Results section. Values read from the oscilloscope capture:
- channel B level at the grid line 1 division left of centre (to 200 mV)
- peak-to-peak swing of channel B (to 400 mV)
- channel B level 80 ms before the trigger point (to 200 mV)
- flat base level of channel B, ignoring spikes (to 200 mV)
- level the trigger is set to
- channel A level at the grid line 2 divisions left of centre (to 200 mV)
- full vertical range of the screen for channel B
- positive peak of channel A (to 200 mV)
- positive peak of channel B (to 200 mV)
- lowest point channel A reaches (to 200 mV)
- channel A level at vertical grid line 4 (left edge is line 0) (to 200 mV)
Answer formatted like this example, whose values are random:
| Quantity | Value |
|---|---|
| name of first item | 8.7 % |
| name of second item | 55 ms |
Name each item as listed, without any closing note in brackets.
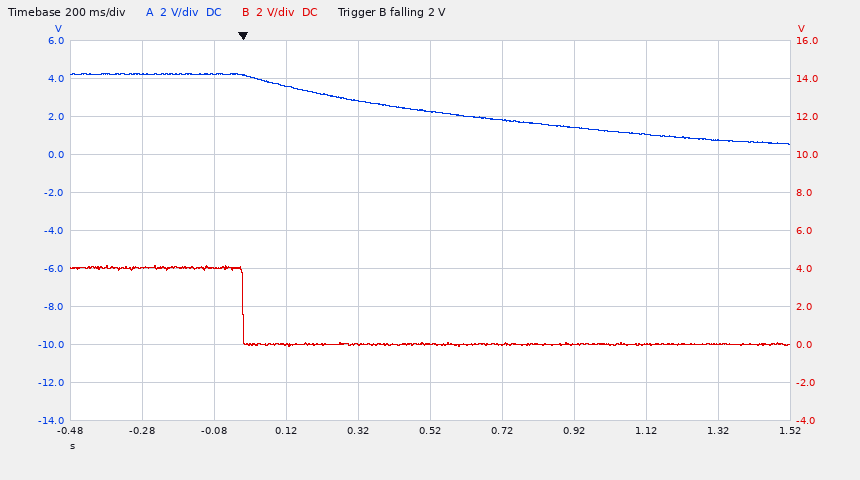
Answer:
| Quantity | Value |
|---|---|
| channel B level at the grid line 1 division left of centre | 0.0 V |
| peak-to-peak swing of channel B | 4.4 V |
| channel B level 80 ms before the trigger point | 4.0 V |
| flat base level of channel B, ignoring spikes | 0.0 V |
| level the trigger is set to | 2 V |
| channel A level at the grid line 2 divisions left of centre | 3.6 V |
| full vertical range of the screen for channel B | 20 V |
| positive peak of channel A | 4.2 V |
| positive peak of channel B | 4.2 V |
| lowest point channel A reaches | 600 mV |
| channel A level at vertical grid line 4 (left edge is line 0) | 2.8 V |
